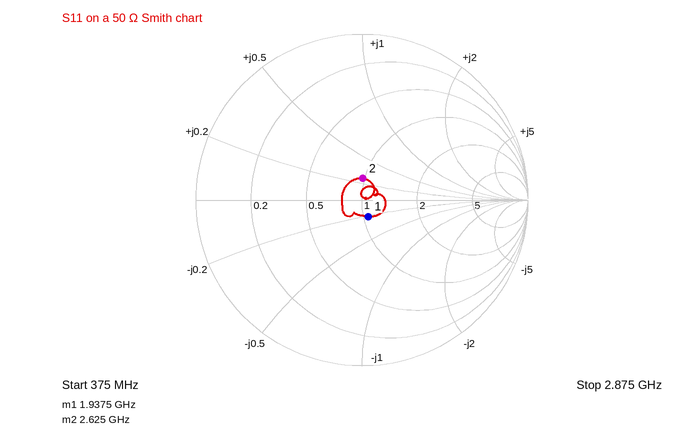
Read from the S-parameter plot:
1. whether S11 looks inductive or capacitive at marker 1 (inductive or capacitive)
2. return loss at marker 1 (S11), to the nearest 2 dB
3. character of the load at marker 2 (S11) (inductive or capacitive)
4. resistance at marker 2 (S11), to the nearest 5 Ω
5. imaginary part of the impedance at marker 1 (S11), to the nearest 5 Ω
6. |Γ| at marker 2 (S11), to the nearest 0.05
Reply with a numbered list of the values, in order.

1. capacitive
2. 20 dB
3. inductive
4. 50 Ω
5. -10 Ω
6. 0.15
